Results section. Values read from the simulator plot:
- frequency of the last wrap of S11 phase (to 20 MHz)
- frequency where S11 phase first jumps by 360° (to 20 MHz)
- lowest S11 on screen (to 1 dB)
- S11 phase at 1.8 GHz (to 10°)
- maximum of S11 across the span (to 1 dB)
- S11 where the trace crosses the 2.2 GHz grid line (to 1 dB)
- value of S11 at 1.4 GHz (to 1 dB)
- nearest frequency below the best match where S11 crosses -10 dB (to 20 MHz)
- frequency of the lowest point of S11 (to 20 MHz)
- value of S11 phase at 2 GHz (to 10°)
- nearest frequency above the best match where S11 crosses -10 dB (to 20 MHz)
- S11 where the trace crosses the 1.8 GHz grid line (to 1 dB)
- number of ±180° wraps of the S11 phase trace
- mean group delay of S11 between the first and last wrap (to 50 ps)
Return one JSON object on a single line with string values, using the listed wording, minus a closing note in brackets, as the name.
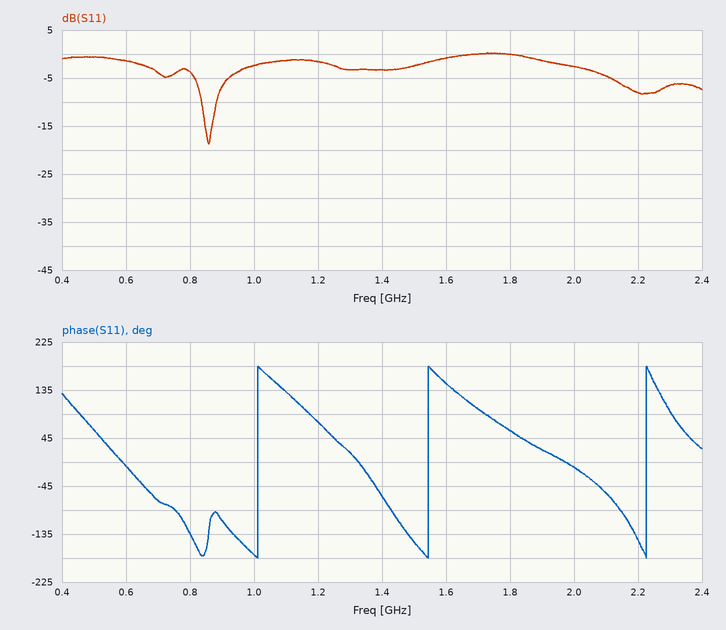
{"frequency of the last wrap of S11 phase": "2.22 GHz", "frequency where S11 phase first jumps by 360°": "1.02 GHz", "lowest S11 on screen": "-19 dB", "S11 phase at 1.8 GHz": "60°", "maximum of S11 across the span": "0 dB", "S11 where the trace crosses the 2.2 GHz grid line": "-8 dB", "value of S11 at 1.4 GHz": "-3 dB", "nearest frequency below the best match where S11 crosses -10 dB": "840 MHz", "frequency of the lowest point of S11": "860 MHz", "value of S11 phase at 2 GHz": "-10°", "nearest frequency above the best match where S11 crosses -10 dB": "880 MHz", "S11 where the trace crosses the 1.8 GHz grid line": "0 dB", "number of ±180° wraps of the S11 phase trace": "3", "mean group delay of S11 between the first and last wrap": "1.65 ns"}
